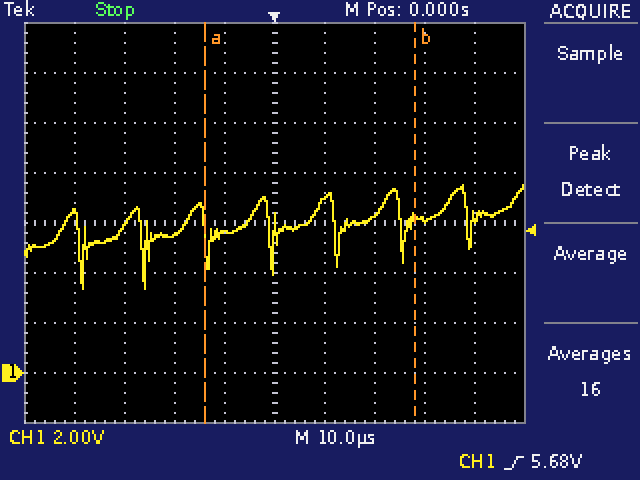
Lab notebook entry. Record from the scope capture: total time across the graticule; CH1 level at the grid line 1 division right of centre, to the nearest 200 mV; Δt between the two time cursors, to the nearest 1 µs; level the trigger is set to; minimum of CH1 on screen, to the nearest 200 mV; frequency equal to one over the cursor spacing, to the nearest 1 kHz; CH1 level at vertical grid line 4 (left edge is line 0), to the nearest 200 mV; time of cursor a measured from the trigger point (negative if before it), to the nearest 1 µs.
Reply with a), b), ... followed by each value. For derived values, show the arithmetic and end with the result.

a) 100 µs
b) 7.0 V
c) 42 µs
d) 5.68 V
e) 3.4 V
f) 1 / 42 µs ≈ 24 kHz
g) 5.6 V
h) -14 µs
